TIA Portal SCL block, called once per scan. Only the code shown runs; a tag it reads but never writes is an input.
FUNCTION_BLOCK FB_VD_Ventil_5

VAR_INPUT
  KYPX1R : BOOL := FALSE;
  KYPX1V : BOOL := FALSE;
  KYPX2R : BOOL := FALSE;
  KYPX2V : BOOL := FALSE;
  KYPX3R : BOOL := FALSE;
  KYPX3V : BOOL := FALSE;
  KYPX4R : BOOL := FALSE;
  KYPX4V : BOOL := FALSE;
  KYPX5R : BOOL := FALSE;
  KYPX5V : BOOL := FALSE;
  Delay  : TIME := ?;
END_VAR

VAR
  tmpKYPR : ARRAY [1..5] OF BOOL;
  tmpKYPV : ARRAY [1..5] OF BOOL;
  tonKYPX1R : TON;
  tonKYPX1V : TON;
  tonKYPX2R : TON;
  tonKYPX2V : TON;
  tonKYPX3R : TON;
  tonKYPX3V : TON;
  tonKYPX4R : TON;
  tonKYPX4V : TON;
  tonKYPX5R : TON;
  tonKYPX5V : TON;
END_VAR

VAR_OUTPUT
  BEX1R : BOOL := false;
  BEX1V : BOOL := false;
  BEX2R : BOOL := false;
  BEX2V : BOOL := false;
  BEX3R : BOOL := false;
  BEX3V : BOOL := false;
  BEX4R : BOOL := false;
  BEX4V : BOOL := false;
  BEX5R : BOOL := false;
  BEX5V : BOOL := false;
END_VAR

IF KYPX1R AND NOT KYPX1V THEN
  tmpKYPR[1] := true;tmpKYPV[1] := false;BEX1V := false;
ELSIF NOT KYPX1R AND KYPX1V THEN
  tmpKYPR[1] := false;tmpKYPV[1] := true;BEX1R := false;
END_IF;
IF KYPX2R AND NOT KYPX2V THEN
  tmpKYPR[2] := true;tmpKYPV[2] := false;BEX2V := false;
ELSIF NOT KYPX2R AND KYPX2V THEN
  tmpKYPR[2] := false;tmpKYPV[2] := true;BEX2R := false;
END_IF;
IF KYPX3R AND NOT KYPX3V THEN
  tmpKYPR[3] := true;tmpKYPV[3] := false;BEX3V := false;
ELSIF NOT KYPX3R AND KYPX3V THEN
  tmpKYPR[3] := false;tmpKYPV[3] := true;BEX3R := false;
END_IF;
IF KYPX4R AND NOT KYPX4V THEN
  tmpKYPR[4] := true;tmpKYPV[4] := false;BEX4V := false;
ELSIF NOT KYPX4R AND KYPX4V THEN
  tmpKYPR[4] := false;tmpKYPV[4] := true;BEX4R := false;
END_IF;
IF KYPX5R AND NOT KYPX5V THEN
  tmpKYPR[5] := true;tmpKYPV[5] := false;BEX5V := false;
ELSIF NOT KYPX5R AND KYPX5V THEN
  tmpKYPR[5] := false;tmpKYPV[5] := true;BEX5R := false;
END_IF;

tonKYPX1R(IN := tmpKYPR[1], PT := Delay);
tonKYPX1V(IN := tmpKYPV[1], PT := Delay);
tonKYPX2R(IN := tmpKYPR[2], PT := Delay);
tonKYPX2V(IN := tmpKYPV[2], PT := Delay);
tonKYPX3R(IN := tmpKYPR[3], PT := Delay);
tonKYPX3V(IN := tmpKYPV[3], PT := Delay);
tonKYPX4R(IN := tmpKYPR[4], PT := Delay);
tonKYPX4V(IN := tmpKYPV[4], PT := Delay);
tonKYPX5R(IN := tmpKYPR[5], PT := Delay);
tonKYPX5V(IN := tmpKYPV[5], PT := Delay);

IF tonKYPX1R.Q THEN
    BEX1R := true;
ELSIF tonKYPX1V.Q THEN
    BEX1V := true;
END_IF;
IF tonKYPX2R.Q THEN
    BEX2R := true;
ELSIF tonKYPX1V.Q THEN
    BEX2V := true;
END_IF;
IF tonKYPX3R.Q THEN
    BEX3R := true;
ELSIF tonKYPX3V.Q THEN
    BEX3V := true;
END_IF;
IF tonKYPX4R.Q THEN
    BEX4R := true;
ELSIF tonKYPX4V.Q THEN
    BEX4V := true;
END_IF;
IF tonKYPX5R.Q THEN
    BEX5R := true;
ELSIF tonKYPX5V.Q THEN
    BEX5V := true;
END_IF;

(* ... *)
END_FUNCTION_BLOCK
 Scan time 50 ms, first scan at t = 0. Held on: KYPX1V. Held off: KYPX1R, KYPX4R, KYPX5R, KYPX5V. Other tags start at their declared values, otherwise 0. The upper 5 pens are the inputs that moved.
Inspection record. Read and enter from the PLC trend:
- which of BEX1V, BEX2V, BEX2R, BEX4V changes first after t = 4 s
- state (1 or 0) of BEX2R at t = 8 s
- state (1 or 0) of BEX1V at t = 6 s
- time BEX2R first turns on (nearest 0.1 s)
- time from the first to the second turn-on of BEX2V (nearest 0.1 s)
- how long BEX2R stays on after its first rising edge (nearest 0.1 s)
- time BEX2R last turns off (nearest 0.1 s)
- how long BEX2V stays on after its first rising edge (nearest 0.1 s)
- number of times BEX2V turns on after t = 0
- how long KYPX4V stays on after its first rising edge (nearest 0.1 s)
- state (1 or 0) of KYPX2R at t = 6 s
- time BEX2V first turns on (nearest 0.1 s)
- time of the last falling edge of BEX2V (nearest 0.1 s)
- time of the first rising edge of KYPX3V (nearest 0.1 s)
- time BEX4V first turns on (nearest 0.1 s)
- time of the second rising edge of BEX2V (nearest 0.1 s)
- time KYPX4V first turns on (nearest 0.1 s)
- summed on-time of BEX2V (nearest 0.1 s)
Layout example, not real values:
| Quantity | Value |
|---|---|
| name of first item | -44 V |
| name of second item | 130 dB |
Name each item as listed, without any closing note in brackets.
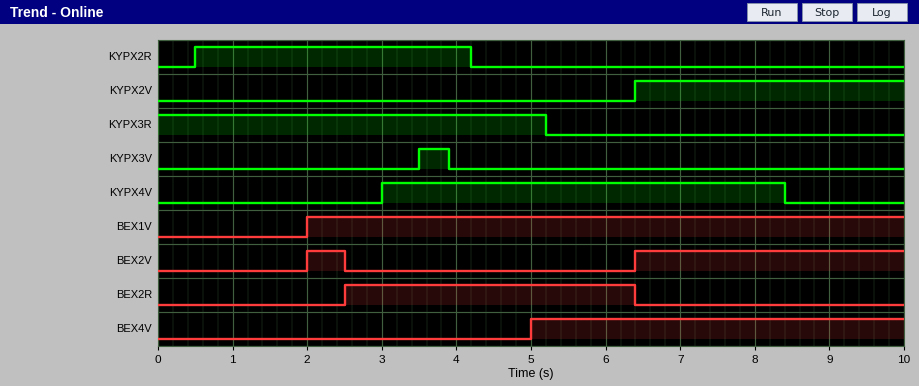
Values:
| Quantity | Value |
|---|---|
| which of BEX1V, BEX2V, BEX2R, BEX4V changes first after t = 4 s | BEX4V |
| state (1 or 0) of BEX2R at t = 8 s | 0 |
| state (1 or 0) of BEX1V at t = 6 s | 1 |
| time BEX2R first turns on | 2.5 s |
| time from the first to the second turn-on of BEX2V | 4.4 s |
| how long BEX2R stays on after its first rising edge | 3.9 s |
| time BEX2R last turns off | 6.4 s |
| how long BEX2V stays on after its first rising edge | 0.5 s |
| number of times BEX2V turns on after t = 0 | 2 |
| how long KYPX4V stays on after its first rising edge | 5.4 s |
| state (1 or 0) of KYPX2R at t = 6 s | 0 |
| time BEX2V first turns on | 2.0 s |
| time of the last falling edge of BEX2V | 2.5 s |
| time of the first rising edge of KYPX3V | 3.5 s |
| time BEX4V first turns on | 5.0 s |
| time of the second rising edge of BEX2V | 6.4 s |
| time KYPX4V first turns on | 3.0 s |
| summed on-time of BEX2V | 4.1 s |
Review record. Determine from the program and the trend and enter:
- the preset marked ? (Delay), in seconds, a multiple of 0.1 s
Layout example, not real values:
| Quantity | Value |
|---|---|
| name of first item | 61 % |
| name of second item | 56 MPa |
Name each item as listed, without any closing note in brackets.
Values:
| Quantity | Value |
|---|---|
| the preset marked ? (Delay), in seconds, a multiple of 0.1 s | 2.0 s |
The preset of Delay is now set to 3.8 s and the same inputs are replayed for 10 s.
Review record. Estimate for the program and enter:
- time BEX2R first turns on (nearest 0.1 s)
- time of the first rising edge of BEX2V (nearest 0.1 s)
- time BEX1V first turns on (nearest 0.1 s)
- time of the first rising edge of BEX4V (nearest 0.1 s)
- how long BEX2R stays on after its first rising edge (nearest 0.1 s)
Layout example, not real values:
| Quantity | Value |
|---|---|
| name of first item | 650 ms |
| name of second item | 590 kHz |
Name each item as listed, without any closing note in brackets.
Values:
| Quantity | Value |
|---|---|
| time BEX2R first turns on | 4.3 s |
| time of the first rising edge of BEX2V | 3.8 s |
| time BEX1V first turns on | 3.8 s |
| time of the first rising edge of BEX4V | 6.8 s |
| how long BEX2R stays on after its first rising edge | 2.1 s |
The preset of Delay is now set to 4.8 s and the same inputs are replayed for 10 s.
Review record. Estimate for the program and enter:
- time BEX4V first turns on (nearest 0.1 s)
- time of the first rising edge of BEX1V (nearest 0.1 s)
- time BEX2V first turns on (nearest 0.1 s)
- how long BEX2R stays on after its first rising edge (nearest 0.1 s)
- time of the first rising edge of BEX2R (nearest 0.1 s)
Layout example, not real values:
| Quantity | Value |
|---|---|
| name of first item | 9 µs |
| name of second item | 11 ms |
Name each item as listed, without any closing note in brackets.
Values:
| Quantity | Value |
|---|---|
| time BEX4V first turns on | 7.8 s |
| time of the first rising edge of BEX1V | 4.8 s |
| time BEX2V first turns on | 4.8 s |
| how long BEX2R stays on after its first rising edge | 1.1 s |
| time of the first rising edge of BEX2R | 5.3 s |
